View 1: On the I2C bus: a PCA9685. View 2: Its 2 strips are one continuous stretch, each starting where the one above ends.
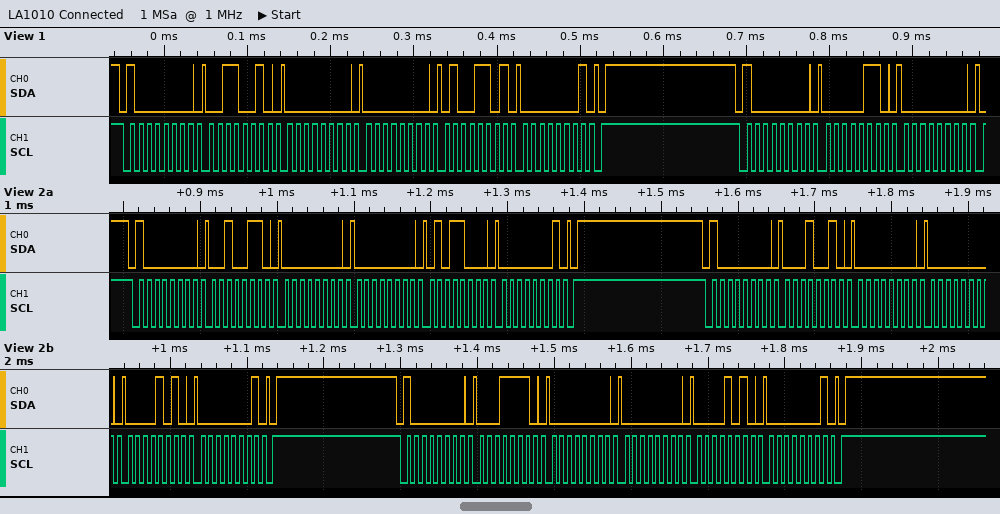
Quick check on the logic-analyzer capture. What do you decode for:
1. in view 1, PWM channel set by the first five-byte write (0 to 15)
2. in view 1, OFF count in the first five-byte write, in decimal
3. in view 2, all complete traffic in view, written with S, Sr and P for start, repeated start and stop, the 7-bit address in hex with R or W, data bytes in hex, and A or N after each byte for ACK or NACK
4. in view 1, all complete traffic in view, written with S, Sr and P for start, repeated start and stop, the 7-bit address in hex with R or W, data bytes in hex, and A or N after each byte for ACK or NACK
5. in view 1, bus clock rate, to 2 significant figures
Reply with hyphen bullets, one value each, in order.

- 11
- 333
- S 40W A 26 A 00 A 00 A 58 A 01 A P S 40W A 12 A 00 A 00 A 0A A 01 A P S 40W A 1E A 00 A 00 A 0A A 01 A P
- S 40W A 32 A 00 A 00 A 4D A 01 A P S 40W A 06 A 00 A
- 100 kHz
